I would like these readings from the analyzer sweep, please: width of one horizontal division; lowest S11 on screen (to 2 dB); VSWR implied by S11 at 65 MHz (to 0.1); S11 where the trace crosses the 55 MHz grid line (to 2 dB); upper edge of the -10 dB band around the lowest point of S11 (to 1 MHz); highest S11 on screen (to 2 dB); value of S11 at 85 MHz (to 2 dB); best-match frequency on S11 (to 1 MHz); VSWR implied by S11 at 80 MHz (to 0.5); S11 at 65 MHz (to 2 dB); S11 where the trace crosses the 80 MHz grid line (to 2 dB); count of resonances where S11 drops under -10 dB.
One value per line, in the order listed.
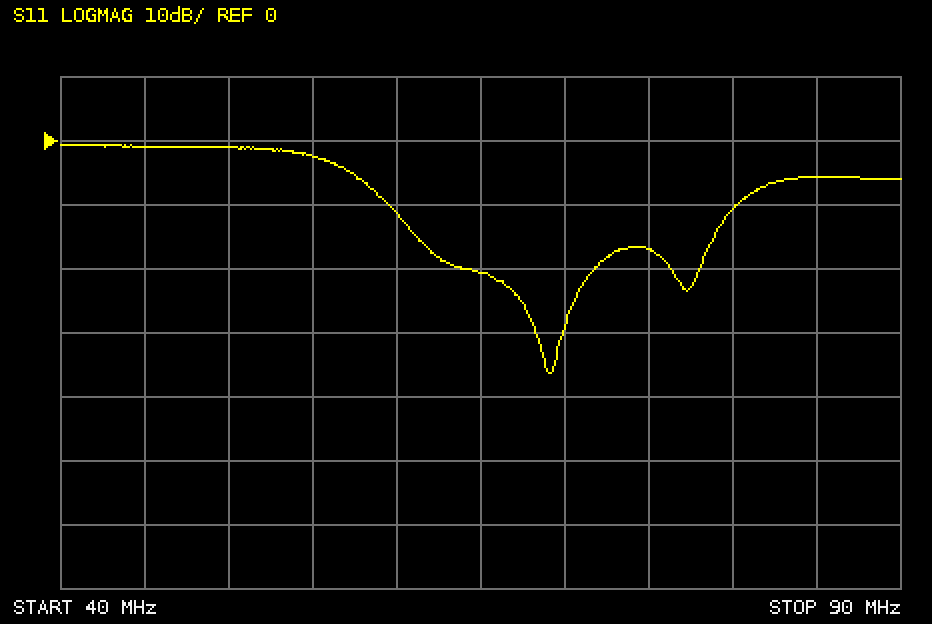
5 MHz
-36 dB
1.2
-2 dB
80 MHz
0 dB
-6 dB
69 MHz
2.0
-20 dB
-10 dB
2
